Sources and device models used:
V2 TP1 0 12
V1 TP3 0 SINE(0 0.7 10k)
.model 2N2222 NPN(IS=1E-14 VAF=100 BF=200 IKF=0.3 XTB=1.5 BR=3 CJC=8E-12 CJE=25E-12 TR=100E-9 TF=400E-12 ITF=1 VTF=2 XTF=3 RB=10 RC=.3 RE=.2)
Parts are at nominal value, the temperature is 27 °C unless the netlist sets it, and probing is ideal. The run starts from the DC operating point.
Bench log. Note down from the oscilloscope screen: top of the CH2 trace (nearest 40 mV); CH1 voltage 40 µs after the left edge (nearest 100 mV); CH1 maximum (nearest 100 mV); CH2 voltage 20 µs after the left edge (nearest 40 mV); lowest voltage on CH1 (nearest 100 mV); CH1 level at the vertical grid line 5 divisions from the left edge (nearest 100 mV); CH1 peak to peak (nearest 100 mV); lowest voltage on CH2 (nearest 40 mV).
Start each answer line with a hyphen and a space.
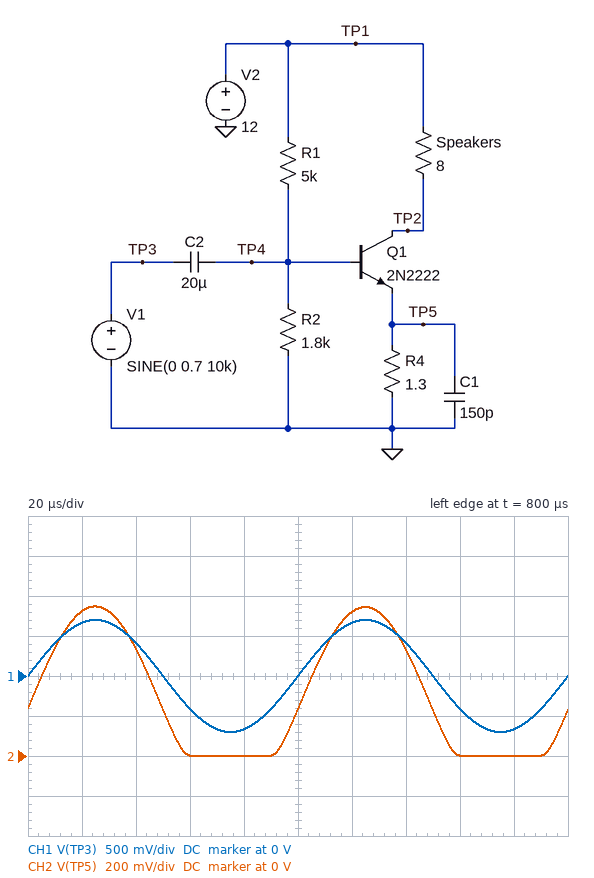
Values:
- 760 mV
- 400 mV
- 700 mV
- 720 mV
- -700 mV
- 0 V
- 1.4 V
- 0 V
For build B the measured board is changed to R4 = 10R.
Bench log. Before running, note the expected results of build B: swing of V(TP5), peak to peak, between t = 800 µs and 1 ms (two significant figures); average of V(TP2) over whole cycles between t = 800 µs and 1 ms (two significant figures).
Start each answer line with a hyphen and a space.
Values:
- 1.3 V
- 11 V
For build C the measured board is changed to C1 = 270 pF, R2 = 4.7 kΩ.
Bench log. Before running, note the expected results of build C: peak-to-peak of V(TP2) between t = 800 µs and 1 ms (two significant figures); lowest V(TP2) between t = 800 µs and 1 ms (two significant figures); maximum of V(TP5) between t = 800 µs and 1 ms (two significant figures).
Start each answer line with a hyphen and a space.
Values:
- 4.8 V
- 7.2 V
- 790 mV
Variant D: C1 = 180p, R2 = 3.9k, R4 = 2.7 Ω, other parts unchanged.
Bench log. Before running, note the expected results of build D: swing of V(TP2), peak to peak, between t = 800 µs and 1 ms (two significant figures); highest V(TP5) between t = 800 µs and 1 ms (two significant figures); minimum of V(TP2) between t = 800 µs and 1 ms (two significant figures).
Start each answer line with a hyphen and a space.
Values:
- 3.4 V
- 1.2 V
- 8.5 V
